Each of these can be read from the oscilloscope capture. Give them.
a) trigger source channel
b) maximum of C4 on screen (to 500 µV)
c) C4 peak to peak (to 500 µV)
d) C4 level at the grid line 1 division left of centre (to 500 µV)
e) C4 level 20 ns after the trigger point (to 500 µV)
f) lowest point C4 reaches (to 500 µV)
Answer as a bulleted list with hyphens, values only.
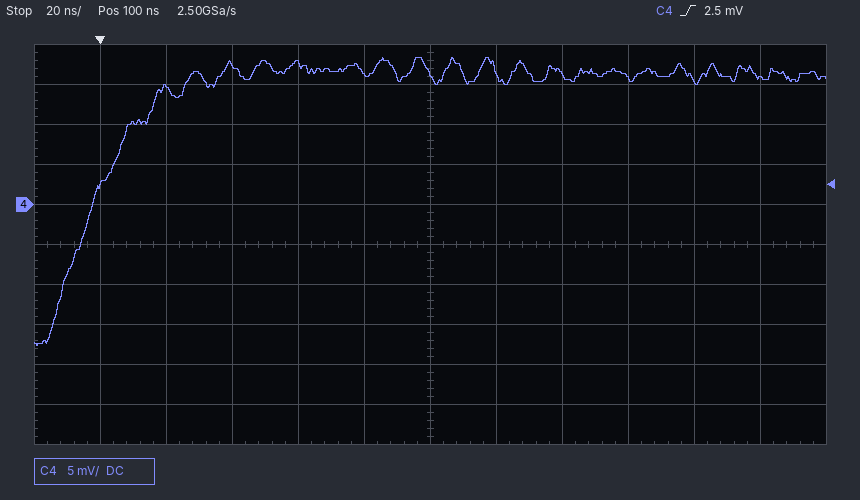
- C4
- 18.5 mV
- 36.0 mV
- 16.5 mV
- 14.5 mV
- -17.5 mV
